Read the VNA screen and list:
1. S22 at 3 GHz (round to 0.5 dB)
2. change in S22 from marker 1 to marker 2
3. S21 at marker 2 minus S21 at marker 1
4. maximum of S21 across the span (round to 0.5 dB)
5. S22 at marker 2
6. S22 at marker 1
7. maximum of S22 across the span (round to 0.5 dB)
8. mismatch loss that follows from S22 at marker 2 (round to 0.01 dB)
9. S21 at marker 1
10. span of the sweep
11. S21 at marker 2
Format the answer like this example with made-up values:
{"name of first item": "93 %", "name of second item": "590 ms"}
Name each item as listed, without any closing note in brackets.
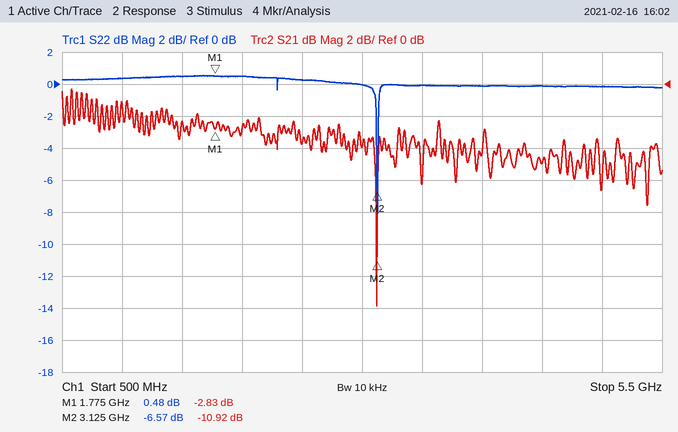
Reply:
{"S22 at 3 GHz": "0.0 dB", "change in S22 from marker 1 to marker 2": "-7.05 dB", "S21 at marker 2 minus S21 at marker 1": "-8.09 dB", "maximum of S21 across the span": "-0.5 dB", "S22 at marker 2": "-6.57 dB", "S22 at marker 1": "0.48 dB", "maximum of S22 across the span": "0.5 dB", "mismatch loss that follows from S22 at marker 2": "1.08 dB", "S21 at marker 1": "-2.83 dB", "span of the sweep": "5 GHz", "S21 at marker 2": "-10.92 dB"}
